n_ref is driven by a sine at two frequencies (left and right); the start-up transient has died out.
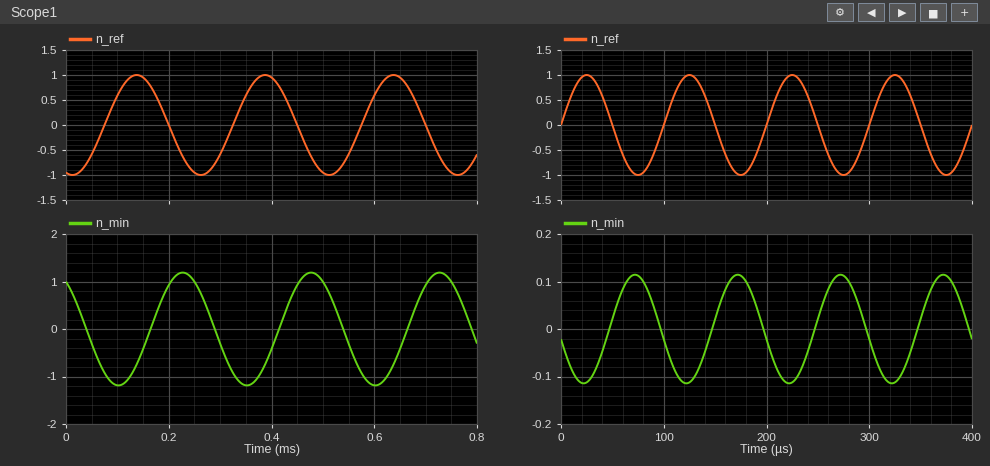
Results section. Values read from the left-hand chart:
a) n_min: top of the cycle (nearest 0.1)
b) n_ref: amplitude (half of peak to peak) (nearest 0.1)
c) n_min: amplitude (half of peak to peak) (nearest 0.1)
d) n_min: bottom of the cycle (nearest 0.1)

1.2
1.0
1.2
-1.2
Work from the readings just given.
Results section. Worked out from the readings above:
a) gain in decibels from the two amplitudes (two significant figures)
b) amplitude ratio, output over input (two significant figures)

1.6 dB
1.2
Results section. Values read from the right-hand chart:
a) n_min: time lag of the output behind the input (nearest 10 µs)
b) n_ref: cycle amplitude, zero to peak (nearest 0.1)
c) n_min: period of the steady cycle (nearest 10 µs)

50 µs
1.0
100 µs
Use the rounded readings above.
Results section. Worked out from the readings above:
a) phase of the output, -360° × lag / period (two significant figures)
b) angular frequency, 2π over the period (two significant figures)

-180°
0.063 rad/µs
